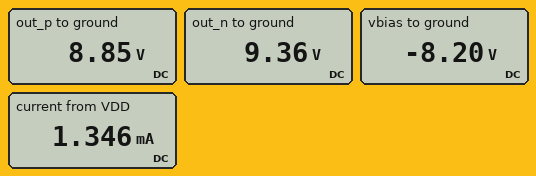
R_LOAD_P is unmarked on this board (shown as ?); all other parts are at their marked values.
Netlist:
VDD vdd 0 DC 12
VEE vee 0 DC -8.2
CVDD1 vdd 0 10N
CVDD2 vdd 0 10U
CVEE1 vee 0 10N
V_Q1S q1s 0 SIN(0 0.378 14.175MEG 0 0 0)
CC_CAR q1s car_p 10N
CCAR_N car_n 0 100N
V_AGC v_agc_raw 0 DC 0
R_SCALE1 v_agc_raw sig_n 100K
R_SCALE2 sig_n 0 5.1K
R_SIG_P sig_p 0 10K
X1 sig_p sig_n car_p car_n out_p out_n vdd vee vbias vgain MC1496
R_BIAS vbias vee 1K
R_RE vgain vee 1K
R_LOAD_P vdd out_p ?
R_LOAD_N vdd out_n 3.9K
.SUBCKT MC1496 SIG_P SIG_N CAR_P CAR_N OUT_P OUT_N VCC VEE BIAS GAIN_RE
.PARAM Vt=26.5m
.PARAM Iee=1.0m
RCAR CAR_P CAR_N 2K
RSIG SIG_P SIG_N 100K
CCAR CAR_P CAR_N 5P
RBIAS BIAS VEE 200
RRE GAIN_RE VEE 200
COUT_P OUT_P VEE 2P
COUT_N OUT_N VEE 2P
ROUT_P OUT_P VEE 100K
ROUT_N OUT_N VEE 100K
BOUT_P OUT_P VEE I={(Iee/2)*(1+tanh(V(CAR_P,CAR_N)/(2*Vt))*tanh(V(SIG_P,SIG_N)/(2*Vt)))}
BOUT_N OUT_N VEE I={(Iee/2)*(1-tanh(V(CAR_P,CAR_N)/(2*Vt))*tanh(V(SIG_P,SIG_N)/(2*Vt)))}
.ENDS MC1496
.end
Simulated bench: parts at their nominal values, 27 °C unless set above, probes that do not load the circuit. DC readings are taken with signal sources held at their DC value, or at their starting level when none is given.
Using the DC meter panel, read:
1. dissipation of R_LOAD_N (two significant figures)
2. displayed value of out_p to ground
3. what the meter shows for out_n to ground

1.8 mW
8.85 V
9.36 V
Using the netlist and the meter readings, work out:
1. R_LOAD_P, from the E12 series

4.7 kΩ
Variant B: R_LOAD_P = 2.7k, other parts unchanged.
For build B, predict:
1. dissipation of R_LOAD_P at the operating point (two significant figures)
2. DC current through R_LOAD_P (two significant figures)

1.3 mW
680 µA
